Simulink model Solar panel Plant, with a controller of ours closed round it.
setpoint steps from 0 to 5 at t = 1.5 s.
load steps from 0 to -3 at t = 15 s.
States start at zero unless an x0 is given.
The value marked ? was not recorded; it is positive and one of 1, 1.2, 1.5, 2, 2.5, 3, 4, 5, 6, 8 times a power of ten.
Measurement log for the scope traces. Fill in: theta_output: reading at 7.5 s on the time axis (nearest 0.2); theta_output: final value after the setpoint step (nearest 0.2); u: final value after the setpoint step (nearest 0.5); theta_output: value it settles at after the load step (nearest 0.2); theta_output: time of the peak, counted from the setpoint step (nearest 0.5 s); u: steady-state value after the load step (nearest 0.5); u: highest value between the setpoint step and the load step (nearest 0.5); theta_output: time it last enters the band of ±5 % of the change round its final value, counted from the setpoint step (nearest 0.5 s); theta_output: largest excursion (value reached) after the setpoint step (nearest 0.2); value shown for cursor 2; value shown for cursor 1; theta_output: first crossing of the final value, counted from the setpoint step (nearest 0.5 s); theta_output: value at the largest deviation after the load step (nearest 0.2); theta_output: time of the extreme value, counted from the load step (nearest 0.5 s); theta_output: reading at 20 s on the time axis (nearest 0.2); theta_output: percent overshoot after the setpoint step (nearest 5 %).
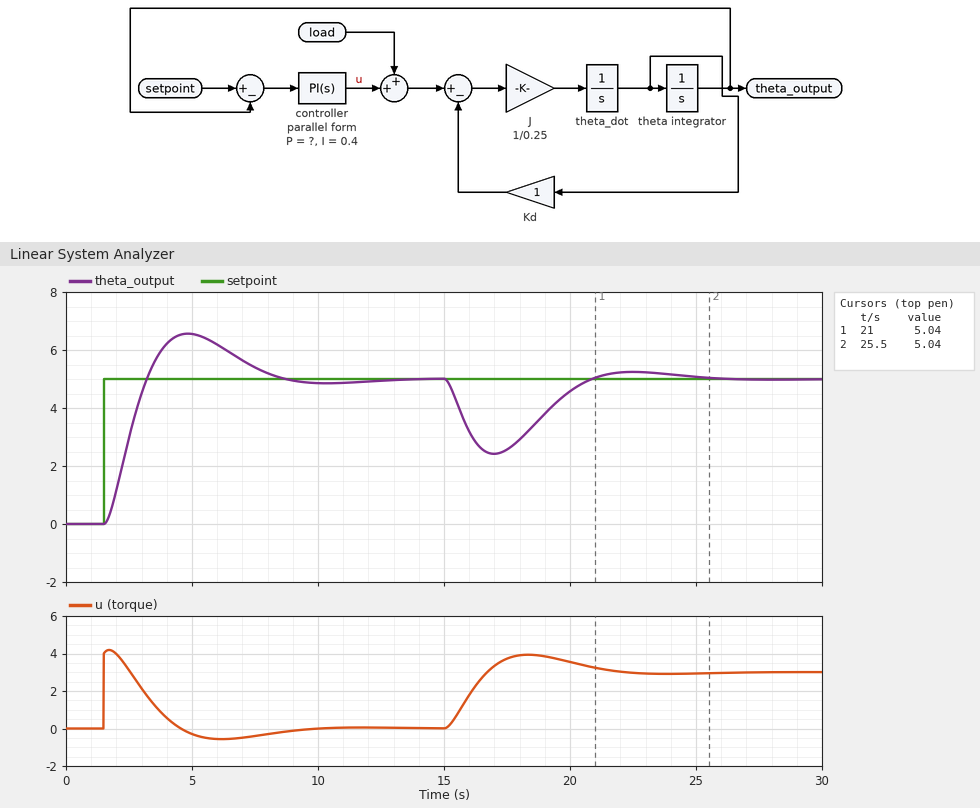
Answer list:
5.4
5.0
0.0
5.0
3.5 s
3.0
4.0
6.5 s
6.6
5.04
5.04
1.5 s
2.4
2.0 s
4.6
30 %
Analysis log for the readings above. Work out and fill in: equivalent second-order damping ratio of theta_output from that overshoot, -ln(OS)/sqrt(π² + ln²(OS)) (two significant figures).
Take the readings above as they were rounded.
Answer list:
0.36
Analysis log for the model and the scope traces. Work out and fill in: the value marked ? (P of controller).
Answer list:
0.8
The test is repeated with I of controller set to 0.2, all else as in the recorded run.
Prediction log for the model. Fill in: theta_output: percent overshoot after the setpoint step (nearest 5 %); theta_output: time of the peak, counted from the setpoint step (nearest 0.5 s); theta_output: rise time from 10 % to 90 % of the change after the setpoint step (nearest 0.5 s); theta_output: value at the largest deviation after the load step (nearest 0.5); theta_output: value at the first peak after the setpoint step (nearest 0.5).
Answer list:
20 %
4.0 s
1.5 s
2.0
6.0
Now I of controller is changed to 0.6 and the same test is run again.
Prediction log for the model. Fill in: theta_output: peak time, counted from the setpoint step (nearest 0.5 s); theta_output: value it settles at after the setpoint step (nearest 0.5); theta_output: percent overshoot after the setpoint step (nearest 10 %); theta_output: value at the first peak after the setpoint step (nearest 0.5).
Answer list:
3.0 s
5.0
40 %
7.0
